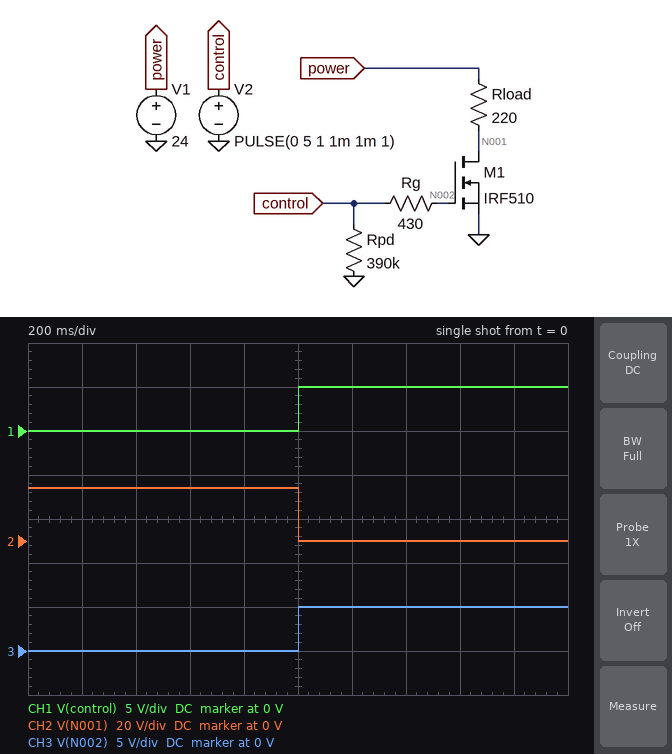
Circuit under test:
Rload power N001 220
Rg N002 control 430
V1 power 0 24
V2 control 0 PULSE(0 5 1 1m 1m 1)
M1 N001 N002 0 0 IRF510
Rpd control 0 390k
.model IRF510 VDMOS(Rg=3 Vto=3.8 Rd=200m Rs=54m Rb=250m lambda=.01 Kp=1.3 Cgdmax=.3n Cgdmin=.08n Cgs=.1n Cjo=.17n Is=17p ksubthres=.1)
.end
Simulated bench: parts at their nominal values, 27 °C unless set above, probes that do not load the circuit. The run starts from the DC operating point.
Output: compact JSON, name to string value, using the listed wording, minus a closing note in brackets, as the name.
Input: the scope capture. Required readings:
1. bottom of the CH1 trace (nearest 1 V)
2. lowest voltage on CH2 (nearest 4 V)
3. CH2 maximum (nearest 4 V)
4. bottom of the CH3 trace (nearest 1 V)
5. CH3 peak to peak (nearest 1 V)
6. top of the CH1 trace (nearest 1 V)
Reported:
{"bottom of the CH1 trace": "0 V", "lowest voltage on CH2": "0 V", "CH2 maximum": "24 V", "bottom of the CH3 trace": "0 V", "CH3 peak to peak": "5 V", "top of the CH1 trace": "5 V"}
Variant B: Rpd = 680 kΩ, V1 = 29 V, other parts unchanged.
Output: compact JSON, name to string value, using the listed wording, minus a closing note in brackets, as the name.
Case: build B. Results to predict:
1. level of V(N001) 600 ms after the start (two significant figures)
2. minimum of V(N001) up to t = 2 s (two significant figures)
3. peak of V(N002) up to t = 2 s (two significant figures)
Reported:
{"level of V(N001) 600 ms after the start": "29 V", "minimum of V(N001) up to t = 2 s": "120 mV", "peak of V(N002) up to t = 2 s": "5.0 V"}
